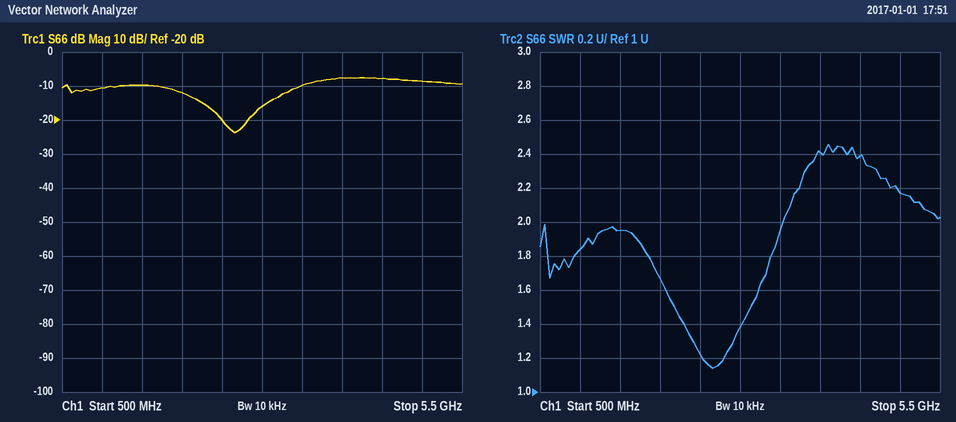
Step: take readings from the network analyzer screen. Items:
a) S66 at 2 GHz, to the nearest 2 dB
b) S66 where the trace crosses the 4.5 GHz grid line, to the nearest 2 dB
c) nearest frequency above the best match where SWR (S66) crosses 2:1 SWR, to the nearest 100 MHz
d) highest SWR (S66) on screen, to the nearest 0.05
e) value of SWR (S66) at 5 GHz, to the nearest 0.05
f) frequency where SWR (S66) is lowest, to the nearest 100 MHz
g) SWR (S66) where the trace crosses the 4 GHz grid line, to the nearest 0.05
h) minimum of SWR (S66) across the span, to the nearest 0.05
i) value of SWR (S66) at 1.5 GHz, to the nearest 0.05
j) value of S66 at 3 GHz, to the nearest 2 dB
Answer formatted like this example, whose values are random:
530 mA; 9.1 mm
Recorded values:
-12 dB; -8 dB; 3.5 GHz; 2.45; 2.15; 2.7 GHz; 2.40; 1.15; 1.95; -16 dB
